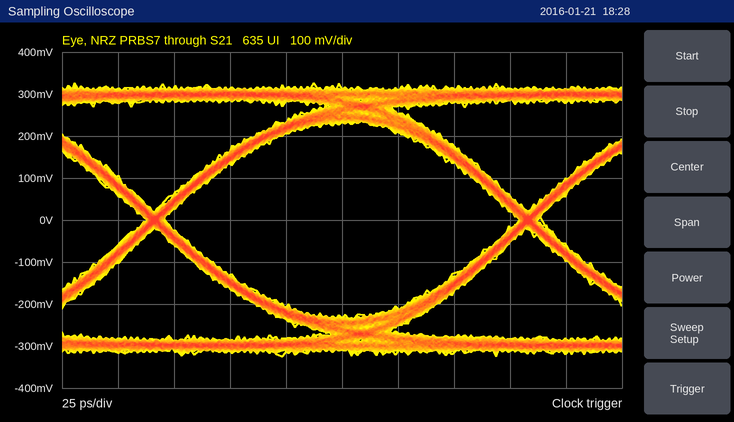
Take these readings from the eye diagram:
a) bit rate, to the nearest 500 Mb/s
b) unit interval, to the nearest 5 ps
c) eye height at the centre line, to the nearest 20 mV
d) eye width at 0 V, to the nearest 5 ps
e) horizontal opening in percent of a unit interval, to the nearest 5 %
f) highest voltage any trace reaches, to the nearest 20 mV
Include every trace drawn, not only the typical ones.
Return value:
6.0 Gb/s
165 ps
460 mV
160 ps
95 %
320 mV
